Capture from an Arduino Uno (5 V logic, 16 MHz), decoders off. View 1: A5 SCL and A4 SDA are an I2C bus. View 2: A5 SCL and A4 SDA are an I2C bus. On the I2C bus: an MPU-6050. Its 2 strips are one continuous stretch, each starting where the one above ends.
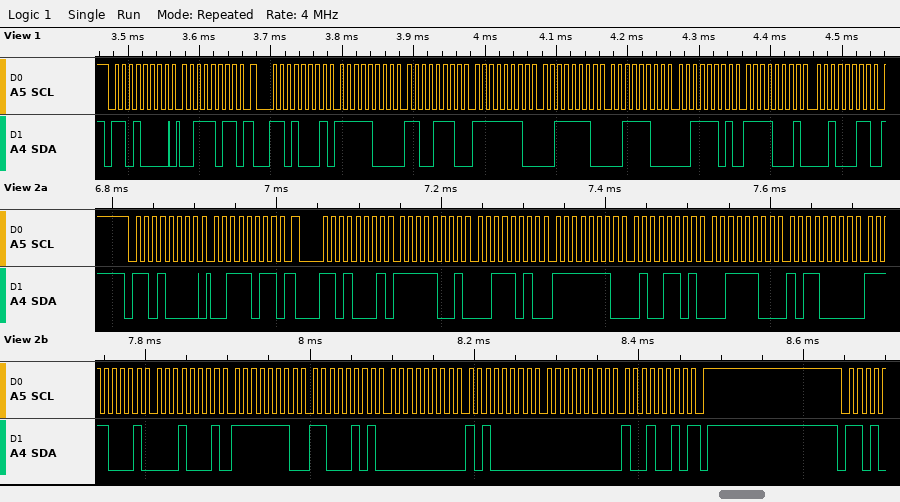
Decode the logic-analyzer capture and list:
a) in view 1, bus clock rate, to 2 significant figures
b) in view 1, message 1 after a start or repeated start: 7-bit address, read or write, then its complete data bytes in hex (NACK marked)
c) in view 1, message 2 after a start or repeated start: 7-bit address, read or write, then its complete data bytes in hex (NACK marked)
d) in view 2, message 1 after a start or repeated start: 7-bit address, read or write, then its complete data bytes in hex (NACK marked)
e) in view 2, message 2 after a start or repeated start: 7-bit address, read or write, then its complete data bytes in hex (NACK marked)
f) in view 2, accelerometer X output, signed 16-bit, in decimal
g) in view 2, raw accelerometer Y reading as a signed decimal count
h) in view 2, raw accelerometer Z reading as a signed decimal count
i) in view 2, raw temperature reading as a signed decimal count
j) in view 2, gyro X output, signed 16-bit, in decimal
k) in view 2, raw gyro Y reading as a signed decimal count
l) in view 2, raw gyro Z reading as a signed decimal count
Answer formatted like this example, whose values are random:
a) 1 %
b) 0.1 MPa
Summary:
a) 100 kHz
b) 0x68 write: 3B
c) 0x68 read: F8 CE FE 3E 3C 3D F1 23
d) 0x68 write: 3B
e) 0x68 read: F9 3A FE 4D 3C B0 F1 11 FE C5 00 A0 00 92 NACK
f) -1734
g) -435
h) 15536
i) -3823
j) -315
k) 160
l) 146
